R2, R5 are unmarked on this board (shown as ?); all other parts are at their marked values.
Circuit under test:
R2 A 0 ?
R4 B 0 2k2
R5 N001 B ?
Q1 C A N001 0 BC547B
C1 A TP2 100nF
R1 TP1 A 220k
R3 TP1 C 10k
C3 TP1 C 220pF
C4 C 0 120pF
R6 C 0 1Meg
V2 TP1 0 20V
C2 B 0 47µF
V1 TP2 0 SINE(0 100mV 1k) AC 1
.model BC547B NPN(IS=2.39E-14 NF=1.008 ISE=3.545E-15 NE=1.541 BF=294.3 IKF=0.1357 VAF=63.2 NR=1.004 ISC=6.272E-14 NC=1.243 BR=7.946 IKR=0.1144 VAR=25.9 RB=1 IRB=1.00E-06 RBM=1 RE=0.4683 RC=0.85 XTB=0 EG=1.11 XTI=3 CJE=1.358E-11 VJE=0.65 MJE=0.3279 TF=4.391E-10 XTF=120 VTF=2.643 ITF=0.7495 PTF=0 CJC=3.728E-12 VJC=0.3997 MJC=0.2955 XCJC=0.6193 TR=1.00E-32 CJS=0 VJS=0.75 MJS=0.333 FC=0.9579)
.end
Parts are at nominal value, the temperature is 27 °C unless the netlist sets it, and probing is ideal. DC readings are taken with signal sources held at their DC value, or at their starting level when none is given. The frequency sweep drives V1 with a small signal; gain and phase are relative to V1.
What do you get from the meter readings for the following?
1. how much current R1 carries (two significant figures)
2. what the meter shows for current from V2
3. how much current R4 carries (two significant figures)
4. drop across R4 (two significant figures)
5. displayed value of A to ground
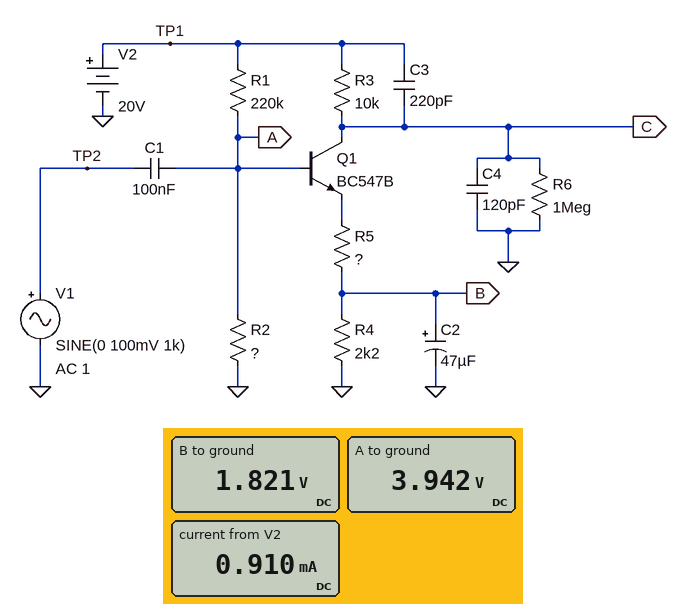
73 µA
0.910 mA
830 µA
1.8 V
3.942 V
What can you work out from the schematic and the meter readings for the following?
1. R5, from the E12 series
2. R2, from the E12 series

1.8 kΩ
56 kΩ
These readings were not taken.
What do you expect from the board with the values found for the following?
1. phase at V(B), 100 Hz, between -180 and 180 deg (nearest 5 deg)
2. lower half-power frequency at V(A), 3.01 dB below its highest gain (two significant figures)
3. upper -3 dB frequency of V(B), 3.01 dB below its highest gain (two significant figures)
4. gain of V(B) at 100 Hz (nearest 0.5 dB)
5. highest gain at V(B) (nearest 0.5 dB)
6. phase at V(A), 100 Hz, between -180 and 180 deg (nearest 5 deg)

-65 deg
39 Hz
45 Hz
-35.5 dB
-27.0 dB
20 deg
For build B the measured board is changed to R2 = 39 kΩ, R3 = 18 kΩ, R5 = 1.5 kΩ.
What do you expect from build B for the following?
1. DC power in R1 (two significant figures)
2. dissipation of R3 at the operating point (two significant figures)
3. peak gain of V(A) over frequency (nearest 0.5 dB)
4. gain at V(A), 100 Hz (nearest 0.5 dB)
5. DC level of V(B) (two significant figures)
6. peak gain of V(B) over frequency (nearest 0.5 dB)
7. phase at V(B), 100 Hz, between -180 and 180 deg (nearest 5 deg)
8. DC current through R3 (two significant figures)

1.3 mW
7.2 mW
0 dB
-1.0 dB
1.4 V
-28.0 dB
-60 deg
630 µA
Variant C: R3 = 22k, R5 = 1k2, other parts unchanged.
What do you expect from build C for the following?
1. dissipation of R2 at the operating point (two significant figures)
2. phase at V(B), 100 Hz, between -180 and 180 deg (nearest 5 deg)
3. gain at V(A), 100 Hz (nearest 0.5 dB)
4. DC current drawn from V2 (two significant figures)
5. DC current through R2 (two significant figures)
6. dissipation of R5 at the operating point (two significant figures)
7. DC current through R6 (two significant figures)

200 µW
-5 deg
-21.0 dB
860 µA
60 µA
760 µW
2.8 µA
